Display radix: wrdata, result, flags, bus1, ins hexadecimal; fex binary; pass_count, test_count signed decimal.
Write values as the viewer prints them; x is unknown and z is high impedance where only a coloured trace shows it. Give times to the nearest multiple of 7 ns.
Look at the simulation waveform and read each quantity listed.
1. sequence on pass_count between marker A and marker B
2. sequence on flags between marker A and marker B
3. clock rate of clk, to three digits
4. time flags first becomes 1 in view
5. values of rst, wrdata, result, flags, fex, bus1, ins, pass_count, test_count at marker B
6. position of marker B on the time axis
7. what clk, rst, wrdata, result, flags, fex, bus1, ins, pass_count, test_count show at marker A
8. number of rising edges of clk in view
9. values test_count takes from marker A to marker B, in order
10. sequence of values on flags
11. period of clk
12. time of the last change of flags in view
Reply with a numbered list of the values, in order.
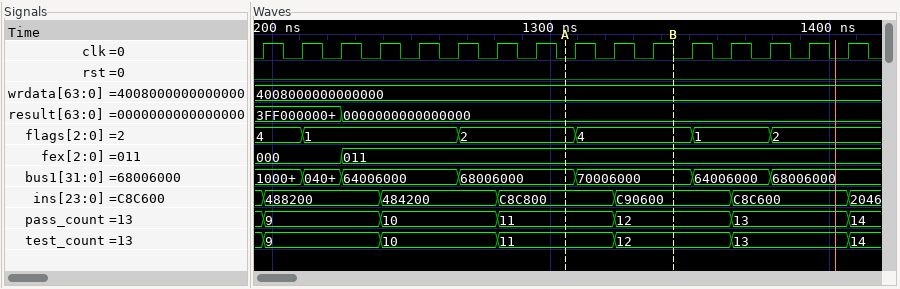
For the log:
1. 11, 12
2. 2, 4
3. 71.4 MHz
4. 1211 ns
5. rst=0, wrdata=4008000000000000, result=0000000000000000, flags=4, fex=011, bus1=70006000, ins=C90600, pass_count=12, test_count=12
6. 1344 ns
7. clk=0, rst=0, wrdata=4008000000000000, result=0000000000000000, flags=2, fex=011, bus1=68006000, ins=C8C800, pass_count=11, test_count=11
8. 16
9. 11, 12
10. 4, 1, 2, 4, 1, 2
11. 14 ns
12. 1379 ns
